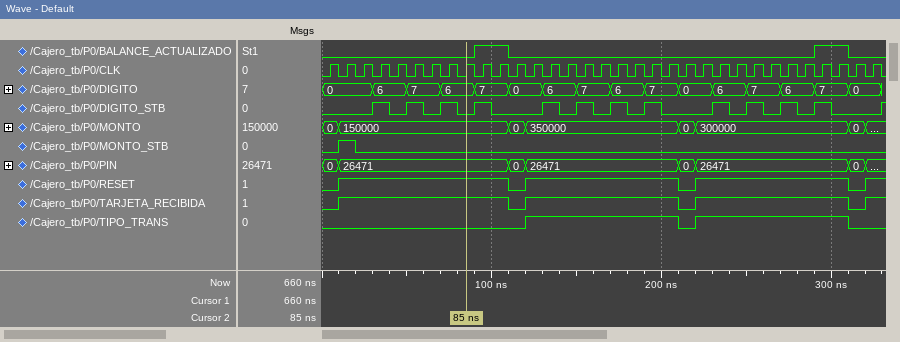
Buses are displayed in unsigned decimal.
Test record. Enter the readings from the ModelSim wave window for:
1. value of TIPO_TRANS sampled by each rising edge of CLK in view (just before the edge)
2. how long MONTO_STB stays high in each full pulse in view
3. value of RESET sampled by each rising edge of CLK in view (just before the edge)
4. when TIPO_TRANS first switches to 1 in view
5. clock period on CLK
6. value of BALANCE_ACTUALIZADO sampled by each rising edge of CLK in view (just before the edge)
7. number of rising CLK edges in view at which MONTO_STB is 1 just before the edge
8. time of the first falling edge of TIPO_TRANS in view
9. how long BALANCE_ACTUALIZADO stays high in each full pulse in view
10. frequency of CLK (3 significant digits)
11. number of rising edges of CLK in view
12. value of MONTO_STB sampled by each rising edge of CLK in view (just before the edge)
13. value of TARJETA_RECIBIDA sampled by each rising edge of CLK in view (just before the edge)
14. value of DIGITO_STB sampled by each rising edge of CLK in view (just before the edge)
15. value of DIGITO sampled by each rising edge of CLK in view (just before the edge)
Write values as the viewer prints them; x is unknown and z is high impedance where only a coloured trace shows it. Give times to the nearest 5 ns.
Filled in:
0 0 0 0 0 0 0 0 0 0 0 0 1 1 1 1 1 1 1 1 1 0 1 1 1 1 1 1 1 1 1 0 0
10 ns
0 1 1 1 1 1 1 1 1 1 1 0 1 1 1 1 1 1 1 1 1 0 1 1 1 1 1 1 1 1 1 0 1
120 ns
10 ns
0 0 0 0 0 0 0 0 0 1 1 0 0 0 0 0 0 0 0 0 0 0 0 0 0 0 0 0 0 1 1 0 0
1
210 ns
20 ns, 20 ns
100 MHz
33
0 1 0 0 0 0 0 0 0 0 0 0 0 0 0 0 0 0 0 0 0 0 0 0 0 0 0 0 0 0 0 0 0
0 1 1 1 1 1 1 1 1 1 1 0 1 1 1 1 1 1 1 1 1 0 1 1 1 1 1 1 1 1 1 0 1
0 0 0 1 0 1 0 1 0 1 0 0 0 1 0 1 0 1 0 1 0 0 0 1 0 1 0 1 0 1 0 0 0
0, 0, 0, 6, 6, 7, 7, 6, 6, 7, 7, 0, 0, 6, 6, 7, 7, 6, 6, 7, 7, 0, 0, 6, 6, 7, 7, 6, 6, 7, 7, 0, 0
